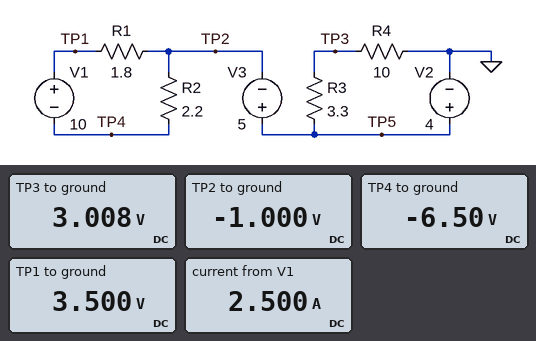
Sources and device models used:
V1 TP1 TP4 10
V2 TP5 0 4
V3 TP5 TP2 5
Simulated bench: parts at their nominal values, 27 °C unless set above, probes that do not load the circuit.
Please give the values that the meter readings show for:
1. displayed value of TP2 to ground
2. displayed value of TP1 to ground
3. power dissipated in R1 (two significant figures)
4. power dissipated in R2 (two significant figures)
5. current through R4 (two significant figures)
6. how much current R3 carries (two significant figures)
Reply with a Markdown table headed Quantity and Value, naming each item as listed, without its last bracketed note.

| Quantity | Value |
|---|---|
| displayed value of TP2 to ground | -1.000 V |
| displayed value of TP1 to ground | 3.500 V |
| power dissipated in R1 | 11 W |
| power dissipated in R2 | 14 W |
| current through R4 | 300 mA |
| how much current R3 carries | 300 mA |
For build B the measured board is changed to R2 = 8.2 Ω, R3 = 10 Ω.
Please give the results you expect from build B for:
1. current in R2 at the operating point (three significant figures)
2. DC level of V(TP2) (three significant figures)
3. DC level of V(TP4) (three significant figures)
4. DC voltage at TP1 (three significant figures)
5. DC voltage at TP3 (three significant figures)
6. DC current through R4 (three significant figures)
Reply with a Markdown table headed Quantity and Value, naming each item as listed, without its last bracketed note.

| Quantity | Value |
|---|---|
| current in R2 at the operating point | 1.00 A |
| DC level of V(TP2) | -1.00 V |
| DC level of V(TP4) | -9.20 V |
| DC voltage at TP1 | 800 mV |
| DC voltage at TP3 | 2.00 V |
| DC current through R4 | 200 mA |
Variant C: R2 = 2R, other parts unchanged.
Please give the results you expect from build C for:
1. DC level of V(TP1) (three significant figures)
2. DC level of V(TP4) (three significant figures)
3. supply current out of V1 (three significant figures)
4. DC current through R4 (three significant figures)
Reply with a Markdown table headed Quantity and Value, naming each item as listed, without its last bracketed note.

| Quantity | Value |
|---|---|
| DC level of V(TP1) | 3.74 V |
| DC level of V(TP4) | -6.26 V |
| supply current out of V1 | 2.63 A |
| DC current through R4 | 301 mA |
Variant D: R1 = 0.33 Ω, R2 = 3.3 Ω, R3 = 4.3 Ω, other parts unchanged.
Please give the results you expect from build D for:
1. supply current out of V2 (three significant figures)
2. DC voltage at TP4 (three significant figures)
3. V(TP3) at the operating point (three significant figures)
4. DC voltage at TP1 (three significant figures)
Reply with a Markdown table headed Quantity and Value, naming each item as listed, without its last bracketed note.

| Quantity | Value |
|---|---|
| supply current out of V2 | 280 mA |
| DC voltage at TP4 | -10.1 V |
| V(TP3) at the operating point | 2.80 V |
| DC voltage at TP1 | -90.9 mV |
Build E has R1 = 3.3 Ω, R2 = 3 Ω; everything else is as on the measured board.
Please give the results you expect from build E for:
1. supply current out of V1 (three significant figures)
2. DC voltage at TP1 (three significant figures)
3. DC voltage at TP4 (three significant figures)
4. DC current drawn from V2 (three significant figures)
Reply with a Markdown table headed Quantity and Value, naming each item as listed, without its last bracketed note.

| Quantity | Value |
|---|---|
| supply current out of V1 | 1.59 A |
| DC voltage at TP1 | 4.24 V |
| DC voltage at TP4 | -5.76 V |
| DC current drawn from V2 | 301 mA |
